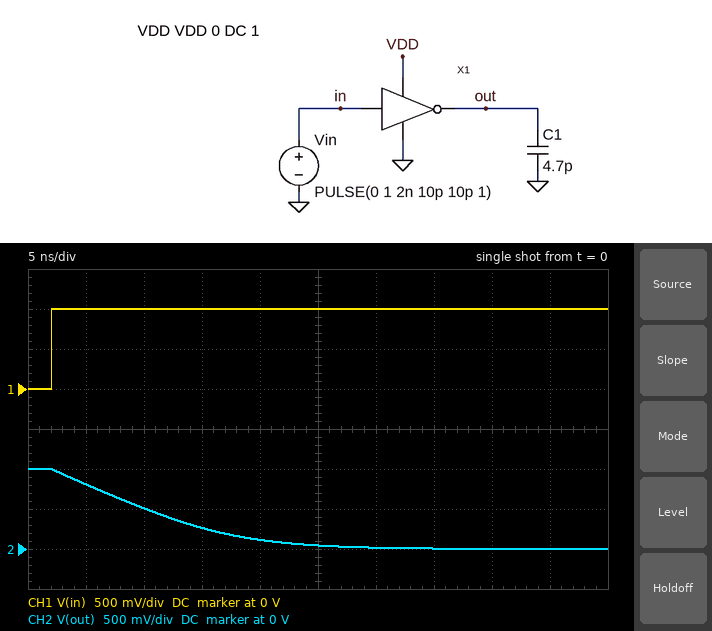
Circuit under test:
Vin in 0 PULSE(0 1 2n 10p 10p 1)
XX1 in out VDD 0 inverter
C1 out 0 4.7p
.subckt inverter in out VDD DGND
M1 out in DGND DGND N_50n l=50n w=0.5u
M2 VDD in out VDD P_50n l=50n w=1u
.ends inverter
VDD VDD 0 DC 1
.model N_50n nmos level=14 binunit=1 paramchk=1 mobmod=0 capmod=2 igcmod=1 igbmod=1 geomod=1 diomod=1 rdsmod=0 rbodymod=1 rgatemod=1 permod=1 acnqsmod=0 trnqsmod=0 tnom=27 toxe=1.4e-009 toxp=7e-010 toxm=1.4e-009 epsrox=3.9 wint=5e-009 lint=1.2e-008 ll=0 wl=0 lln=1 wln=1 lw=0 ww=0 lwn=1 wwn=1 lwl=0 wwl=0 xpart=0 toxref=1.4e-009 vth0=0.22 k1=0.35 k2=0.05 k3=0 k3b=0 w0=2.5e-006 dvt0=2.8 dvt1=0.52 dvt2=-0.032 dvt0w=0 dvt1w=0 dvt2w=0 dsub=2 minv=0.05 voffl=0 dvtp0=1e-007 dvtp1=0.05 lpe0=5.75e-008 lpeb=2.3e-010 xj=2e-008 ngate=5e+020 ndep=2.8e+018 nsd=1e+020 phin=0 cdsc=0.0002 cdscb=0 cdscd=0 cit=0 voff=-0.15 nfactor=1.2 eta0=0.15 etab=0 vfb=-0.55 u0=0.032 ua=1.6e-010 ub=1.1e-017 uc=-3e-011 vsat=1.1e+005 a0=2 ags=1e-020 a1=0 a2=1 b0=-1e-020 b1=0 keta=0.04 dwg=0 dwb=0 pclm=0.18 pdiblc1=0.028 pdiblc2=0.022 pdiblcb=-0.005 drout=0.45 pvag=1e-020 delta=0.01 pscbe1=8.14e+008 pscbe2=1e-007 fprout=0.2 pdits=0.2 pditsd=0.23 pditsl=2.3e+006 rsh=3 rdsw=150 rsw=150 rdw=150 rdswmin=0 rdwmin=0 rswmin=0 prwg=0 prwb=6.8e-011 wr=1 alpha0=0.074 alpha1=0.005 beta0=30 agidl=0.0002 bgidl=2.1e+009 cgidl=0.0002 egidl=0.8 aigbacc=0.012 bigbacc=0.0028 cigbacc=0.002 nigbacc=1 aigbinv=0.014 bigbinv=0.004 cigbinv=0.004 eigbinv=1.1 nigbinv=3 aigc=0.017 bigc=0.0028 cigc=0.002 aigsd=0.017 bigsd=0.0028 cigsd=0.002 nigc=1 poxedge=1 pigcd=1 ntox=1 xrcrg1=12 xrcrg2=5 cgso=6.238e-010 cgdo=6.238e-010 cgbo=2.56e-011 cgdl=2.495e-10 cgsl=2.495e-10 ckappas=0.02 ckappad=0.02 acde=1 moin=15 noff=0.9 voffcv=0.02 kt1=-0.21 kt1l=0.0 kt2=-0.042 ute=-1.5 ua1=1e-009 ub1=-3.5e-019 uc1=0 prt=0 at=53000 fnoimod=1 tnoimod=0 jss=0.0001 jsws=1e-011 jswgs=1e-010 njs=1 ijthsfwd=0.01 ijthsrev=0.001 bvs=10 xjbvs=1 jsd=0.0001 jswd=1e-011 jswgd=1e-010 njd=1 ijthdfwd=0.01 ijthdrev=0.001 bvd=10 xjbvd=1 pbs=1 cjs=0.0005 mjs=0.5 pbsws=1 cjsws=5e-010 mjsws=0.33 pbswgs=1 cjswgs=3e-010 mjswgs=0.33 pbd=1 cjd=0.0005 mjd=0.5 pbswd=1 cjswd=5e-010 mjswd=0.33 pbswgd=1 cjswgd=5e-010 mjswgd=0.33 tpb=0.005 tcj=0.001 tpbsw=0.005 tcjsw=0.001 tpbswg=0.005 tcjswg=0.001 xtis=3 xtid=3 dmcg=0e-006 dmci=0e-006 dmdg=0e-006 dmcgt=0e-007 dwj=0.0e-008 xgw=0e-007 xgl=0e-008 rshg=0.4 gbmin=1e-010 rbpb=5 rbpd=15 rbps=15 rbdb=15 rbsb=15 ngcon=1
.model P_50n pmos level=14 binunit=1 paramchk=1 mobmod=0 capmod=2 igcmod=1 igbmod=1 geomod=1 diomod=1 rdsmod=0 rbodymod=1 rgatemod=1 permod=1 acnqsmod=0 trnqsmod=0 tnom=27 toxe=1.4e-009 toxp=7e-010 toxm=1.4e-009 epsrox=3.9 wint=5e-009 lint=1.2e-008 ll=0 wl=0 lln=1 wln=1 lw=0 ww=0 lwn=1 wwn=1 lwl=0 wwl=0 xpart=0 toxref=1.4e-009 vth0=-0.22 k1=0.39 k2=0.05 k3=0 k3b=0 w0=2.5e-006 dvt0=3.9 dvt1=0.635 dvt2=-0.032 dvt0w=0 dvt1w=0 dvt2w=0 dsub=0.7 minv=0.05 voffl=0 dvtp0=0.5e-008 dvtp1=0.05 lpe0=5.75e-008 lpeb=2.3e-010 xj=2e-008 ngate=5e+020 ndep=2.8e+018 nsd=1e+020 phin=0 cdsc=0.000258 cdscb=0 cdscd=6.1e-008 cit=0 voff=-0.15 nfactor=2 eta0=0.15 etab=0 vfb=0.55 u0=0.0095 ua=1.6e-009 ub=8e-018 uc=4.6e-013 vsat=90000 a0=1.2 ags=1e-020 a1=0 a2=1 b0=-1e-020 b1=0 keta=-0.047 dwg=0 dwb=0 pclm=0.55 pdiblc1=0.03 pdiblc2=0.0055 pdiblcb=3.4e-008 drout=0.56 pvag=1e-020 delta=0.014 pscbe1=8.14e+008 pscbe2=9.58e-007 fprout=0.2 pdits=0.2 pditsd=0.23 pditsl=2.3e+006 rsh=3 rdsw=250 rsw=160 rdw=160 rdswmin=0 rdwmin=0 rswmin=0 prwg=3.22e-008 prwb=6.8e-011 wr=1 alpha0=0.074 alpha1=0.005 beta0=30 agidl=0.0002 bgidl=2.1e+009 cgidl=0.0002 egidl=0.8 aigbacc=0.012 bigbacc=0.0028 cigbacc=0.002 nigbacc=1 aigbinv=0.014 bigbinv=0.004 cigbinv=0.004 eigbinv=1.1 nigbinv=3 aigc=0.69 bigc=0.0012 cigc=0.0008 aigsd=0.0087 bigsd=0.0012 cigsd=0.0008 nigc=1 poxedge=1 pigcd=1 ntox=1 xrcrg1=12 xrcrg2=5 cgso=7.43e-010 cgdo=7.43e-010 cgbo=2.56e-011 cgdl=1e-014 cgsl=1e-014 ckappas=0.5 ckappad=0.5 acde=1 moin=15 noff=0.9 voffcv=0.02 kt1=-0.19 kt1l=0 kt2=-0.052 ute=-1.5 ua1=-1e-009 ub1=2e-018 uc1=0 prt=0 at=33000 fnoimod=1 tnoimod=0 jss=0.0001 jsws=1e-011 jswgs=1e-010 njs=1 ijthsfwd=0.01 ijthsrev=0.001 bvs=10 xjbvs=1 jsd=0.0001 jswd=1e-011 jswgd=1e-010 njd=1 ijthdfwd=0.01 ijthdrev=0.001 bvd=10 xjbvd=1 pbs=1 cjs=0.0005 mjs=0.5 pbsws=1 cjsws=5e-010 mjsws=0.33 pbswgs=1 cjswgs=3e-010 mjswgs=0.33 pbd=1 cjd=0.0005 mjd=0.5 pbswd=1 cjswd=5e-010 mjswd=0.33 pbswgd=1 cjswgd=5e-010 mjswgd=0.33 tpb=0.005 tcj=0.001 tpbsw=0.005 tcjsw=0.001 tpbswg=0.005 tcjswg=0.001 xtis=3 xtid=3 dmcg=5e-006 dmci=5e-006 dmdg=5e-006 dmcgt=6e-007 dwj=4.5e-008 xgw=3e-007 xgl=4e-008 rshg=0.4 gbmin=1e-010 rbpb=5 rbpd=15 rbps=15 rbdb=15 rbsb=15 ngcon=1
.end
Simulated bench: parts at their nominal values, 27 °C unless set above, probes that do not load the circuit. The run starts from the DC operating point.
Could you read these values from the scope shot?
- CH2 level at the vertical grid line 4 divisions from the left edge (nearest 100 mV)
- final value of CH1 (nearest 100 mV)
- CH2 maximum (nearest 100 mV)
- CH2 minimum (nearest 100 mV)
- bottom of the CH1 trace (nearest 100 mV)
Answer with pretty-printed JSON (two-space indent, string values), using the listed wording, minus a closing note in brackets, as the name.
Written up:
{
  "CH2 level at the vertical grid line 4 divisions from the left edge": "100 mV",
  "final value of CH1": "1.0 V",
  "CH2 maximum": "1.0 V",
  "CH2 minimum": "0 V",
  "bottom of the CH1 trace": "0 V"
}
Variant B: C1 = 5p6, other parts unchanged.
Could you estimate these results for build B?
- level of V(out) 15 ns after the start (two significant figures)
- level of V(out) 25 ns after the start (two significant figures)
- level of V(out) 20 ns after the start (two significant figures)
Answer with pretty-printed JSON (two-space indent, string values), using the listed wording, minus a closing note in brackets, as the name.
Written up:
{
  "level of V(out) 15 ns after the start": "360 mV",
  "level of V(out) 25 ns after the start": "89 mV",
  "level of V(out) 20 ns after the start": "190 mV"
}
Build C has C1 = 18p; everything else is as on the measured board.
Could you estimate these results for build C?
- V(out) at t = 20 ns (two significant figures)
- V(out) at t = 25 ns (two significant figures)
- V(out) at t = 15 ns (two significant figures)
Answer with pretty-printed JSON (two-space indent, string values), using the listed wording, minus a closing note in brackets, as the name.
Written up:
{
  "V(out) at t = 20 ns": "700 mV",
  "V(out) at t = 25 ns": "620 mV",
  "V(out) at t = 15 ns": "780 mV"
}
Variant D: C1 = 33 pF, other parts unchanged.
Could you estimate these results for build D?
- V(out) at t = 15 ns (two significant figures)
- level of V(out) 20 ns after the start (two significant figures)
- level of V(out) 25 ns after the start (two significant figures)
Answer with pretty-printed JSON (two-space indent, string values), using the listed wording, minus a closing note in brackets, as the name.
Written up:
{
  "V(out) at t = 15 ns": "880 mV",
  "level of V(out) 20 ns after the start": "830 mV",
  "level of V(out) 25 ns after the start": "790 mV"
}
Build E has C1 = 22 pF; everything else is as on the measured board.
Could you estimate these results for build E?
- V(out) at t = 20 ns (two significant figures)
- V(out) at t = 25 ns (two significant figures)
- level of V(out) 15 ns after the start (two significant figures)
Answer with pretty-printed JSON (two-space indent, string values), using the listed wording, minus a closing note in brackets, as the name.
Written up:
{
  "V(out) at t = 20 ns": "750 mV",
  "V(out) at t = 25 ns": "690 mV",
  "level of V(out) 15 ns after the start": "820 mV"
}
